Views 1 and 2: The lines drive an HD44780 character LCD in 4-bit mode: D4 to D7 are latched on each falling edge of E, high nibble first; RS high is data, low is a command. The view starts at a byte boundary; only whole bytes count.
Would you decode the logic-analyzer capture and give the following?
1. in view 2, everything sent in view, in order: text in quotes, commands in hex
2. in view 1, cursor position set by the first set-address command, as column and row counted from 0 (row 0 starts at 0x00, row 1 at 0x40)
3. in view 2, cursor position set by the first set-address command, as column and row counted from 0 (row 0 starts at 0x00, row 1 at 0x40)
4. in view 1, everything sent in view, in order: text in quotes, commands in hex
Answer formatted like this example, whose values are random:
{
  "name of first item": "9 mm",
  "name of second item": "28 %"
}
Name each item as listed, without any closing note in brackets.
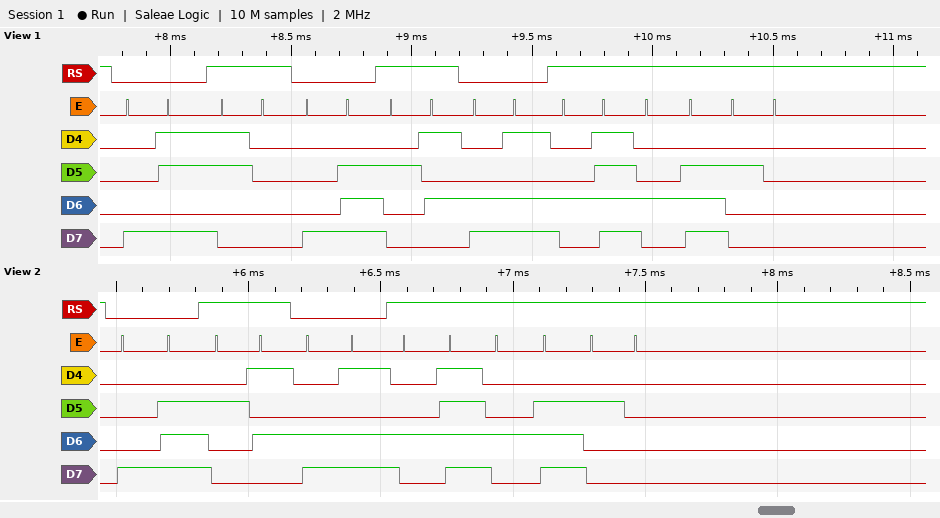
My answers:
{
  "in view 2, everything sent in view, in order: text in quotes, commands in hex": "0x8E \"%\" 0xCD \"ON \"",
  "in view 1, cursor position set by the first set-address command, as column and row counted from 0": "column 11, row 0",
  "in view 2, cursor position set by the first set-address command, as column and row counted from 0": "column 14, row 0",
  "in view 1, everything sent in view, in order: text in quotes, commands in hex": "0x8B \"0\" 0x8E \"%\" 0xCD \"ON \""
}
